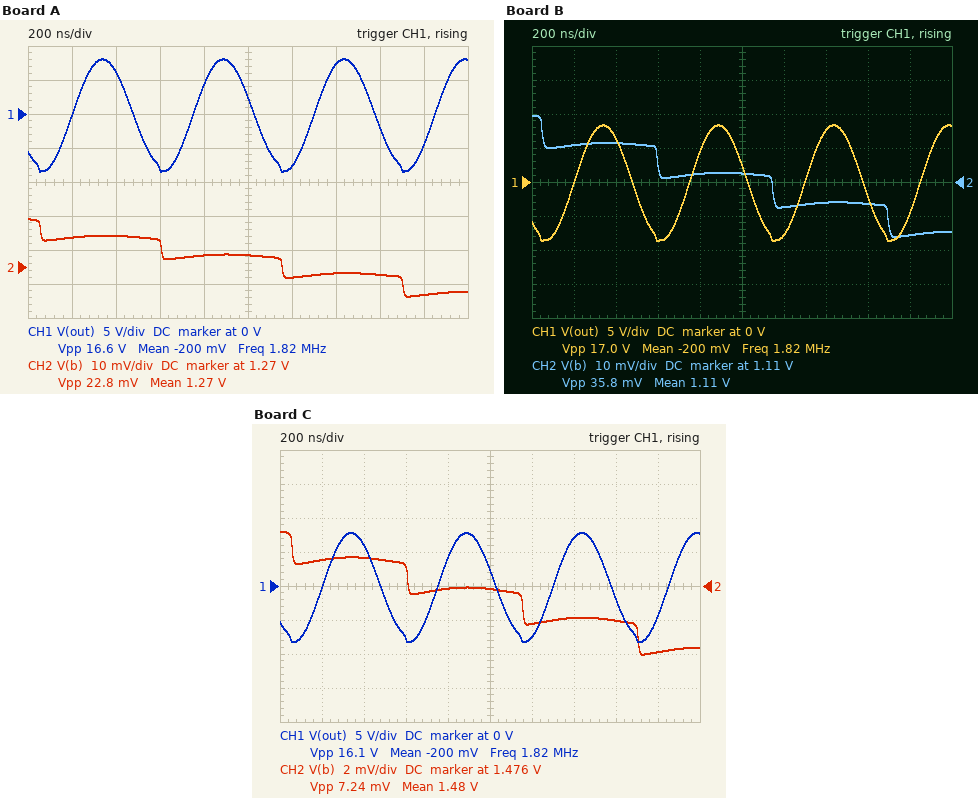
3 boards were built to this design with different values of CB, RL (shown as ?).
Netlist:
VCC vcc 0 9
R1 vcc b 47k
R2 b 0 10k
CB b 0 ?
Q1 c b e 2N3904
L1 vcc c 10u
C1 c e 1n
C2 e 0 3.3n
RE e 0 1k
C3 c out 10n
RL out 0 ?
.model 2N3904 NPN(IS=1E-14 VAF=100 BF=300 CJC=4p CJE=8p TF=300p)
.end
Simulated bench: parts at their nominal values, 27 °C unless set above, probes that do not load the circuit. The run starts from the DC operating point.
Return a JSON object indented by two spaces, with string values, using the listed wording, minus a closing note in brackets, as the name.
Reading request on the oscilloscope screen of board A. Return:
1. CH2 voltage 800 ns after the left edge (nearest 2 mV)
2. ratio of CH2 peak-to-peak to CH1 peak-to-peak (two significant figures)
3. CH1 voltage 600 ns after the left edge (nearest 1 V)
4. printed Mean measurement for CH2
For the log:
{
  "CH2 voltage 800 ns after the left edge": "1.274 V",
  "ratio of CH2 peak-to-peak to CH1 peak-to-peak": "0.0014",
  "CH1 voltage 600 ns after the left edge": "-8 V",
  "printed Mean measurement for CH2": "1.27 V"
}
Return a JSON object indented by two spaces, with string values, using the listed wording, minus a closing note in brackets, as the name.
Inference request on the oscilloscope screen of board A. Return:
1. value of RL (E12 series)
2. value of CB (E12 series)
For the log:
{
  "value of RL": "3.9 kΩ",
  "value of CB": "47 nF"
}
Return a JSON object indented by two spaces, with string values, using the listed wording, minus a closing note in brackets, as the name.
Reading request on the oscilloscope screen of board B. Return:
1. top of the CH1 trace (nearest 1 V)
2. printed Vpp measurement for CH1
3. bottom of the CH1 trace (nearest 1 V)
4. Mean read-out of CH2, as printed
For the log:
{
  "top of the CH1 trace": "8 V",
  "printed Vpp measurement for CH1": "17.0 V",
  "bottom of the CH1 trace": "-9 V",
  "Mean read-out of CH2, as printed": "1.11 V"
}
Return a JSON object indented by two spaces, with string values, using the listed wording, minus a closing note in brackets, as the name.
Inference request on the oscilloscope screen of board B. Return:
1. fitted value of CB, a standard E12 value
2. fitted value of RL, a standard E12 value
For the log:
{
  "fitted value of CB, a standard E12 value": "47 nF",
  "fitted value of RL, a standard E12 value": "6.8 kΩ"
}
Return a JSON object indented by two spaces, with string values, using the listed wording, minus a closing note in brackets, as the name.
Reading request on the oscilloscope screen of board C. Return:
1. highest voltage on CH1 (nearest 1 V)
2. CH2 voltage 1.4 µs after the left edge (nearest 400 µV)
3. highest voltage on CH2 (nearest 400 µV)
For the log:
{
  "highest voltage on CH1": "8 V",
  "CH2 voltage 1.4 µs after the left edge": "1.4740 V",
  "highest voltage on CH2": "1.4792 V"
}
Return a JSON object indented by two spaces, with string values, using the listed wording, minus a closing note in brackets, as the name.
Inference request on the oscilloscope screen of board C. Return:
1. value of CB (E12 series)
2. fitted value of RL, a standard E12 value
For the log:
{
  "value of CB": "150 nF",
  "fitted value of RL, a standard E12 value": "3.3 kΩ"
}
